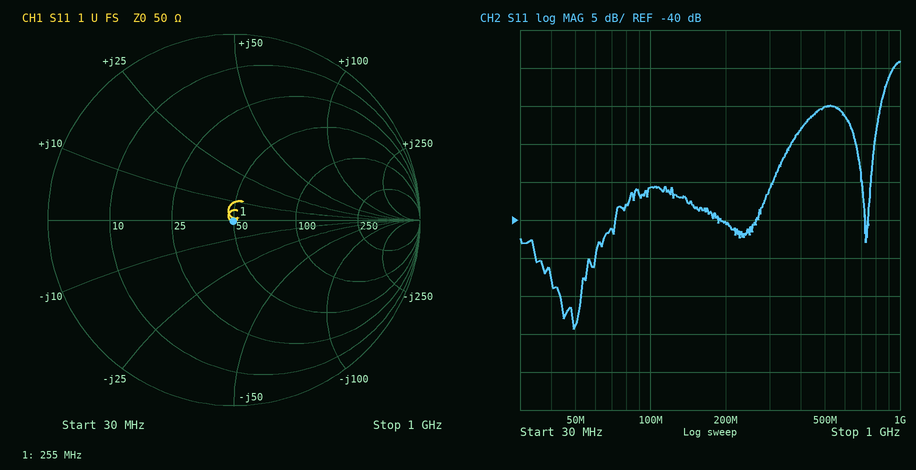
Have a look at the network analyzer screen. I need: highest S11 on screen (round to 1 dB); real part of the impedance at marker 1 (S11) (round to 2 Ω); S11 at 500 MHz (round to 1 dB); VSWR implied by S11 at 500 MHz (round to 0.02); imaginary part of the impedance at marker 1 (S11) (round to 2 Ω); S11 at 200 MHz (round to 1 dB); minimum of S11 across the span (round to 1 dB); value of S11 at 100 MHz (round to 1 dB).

-19 dB
50 Ω
-25 dB
1.12
0 Ω
-40 dB
-54 dB
-36 dB
